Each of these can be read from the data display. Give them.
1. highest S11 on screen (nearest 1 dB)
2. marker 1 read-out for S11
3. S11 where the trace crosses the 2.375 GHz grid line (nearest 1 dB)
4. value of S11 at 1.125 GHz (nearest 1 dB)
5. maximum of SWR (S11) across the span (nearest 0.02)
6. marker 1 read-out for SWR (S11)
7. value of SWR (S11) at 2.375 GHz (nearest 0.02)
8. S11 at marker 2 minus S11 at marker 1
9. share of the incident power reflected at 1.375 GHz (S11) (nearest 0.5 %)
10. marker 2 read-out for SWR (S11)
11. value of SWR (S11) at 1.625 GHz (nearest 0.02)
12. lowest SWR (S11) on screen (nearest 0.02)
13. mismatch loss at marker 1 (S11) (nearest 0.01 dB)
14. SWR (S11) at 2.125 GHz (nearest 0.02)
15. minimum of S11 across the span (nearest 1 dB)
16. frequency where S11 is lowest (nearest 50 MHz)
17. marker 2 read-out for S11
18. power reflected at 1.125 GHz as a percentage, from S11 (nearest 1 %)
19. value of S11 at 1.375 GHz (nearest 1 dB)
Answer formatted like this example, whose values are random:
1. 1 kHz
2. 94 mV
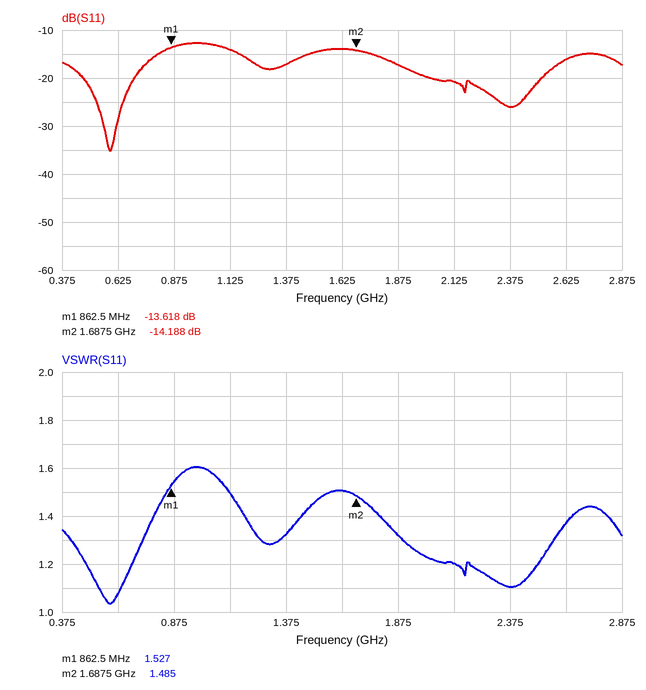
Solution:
1. -13 dB
2. -13.618 dB
3. -26 dB
4. -14 dB
5. 1.60
6. 1.527
7. 1.10
8. -0.570 dB
9. 2.0 %
10. 1.485
11. 1.50
12. 1.04
13. 0.19 dB
14. 1.20
15. -35 dB
16. 600 MHz
17. -14.188 dB
18. 4 %
19. -17 dB
